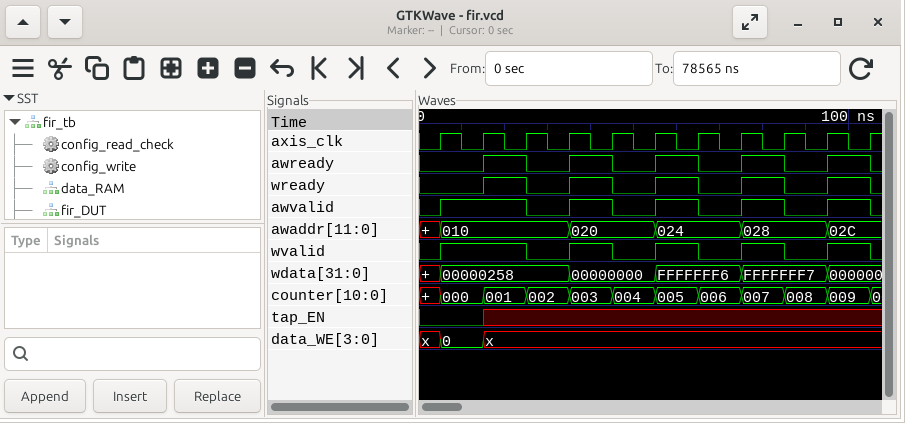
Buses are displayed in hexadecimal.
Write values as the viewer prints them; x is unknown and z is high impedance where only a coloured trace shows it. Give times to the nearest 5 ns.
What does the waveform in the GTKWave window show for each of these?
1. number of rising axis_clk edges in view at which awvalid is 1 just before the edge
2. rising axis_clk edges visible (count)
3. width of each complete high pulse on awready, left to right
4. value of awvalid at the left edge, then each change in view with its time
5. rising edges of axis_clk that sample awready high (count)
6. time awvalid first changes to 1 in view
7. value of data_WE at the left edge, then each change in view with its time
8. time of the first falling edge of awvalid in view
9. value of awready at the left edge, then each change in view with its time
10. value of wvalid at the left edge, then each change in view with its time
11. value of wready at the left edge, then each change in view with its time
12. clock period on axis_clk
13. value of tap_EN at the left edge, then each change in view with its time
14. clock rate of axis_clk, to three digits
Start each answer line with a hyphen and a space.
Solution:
- 6
- 11
- 10 ns, 10 ns, 10 ns, 10 ns, 10 ns
- 0, 1 at 5 ns, 0 at 25 ns, 1 at 35 ns, 0 at 45 ns, 1 at 55 ns, 0 at 65 ns, 1 at 75 ns, 0 at 85 ns, 1 at 95 ns, 0 at 105 ns
- 5
- 5 ns
- x, 0 at 5 ns, x at 15 ns
- 25 ns
- 0, 1 at 15 ns, 0 at 25 ns, 1 at 35 ns, 0 at 45 ns, 1 at 55 ns, 0 at 65 ns, 1 at 75 ns, 0 at 85 ns, 1 at 95 ns, 0 at 105 ns
- 0, 1 at 5 ns, 0 at 25 ns, 1 at 35 ns, 0 at 45 ns, 1 at 55 ns, 0 at 65 ns, 1 at 75 ns, 0 at 85 ns, 1 at 95 ns, 0 at 105 ns
- 0, 1 at 15 ns, 0 at 25 ns, 1 at 35 ns, 0 at 45 ns, 1 at 55 ns, 0 at 65 ns, 1 at 75 ns, 0 at 85 ns, 1 at 95 ns, 0 at 105 ns
- 10 ns
- 0, x at 15 ns
- 100 MHz
